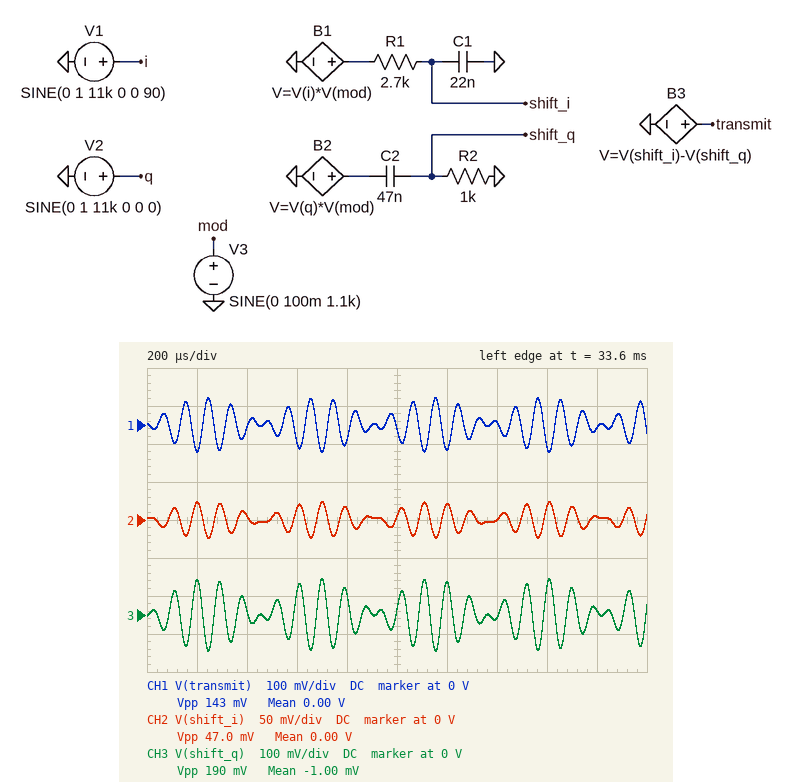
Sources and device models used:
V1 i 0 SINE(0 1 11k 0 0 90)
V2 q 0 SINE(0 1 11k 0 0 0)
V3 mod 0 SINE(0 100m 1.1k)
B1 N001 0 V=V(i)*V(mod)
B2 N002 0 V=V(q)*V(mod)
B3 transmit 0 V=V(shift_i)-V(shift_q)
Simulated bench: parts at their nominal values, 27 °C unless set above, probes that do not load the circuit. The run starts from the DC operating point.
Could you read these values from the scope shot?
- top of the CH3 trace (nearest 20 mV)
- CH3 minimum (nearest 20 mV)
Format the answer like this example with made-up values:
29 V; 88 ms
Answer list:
100 mV; -100 mV
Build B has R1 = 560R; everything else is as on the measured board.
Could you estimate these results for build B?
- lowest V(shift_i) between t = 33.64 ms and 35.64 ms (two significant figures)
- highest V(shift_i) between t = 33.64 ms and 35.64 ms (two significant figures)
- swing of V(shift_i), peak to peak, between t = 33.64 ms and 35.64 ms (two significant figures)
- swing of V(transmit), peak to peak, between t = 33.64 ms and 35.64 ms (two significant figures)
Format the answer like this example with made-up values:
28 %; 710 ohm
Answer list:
-76 mV; 76 mV; 150 mV; 100 mV
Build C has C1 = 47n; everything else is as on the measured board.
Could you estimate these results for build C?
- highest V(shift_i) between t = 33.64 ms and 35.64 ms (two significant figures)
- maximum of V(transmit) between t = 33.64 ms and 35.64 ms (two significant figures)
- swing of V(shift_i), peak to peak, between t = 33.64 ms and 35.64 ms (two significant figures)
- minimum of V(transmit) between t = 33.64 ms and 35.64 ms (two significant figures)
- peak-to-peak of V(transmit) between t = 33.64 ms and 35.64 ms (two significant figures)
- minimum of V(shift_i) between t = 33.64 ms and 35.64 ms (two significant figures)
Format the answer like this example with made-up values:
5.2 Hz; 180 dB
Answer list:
11 mV; 84 mV; 23 mV; -84 mV; 170 mV; -11 mV
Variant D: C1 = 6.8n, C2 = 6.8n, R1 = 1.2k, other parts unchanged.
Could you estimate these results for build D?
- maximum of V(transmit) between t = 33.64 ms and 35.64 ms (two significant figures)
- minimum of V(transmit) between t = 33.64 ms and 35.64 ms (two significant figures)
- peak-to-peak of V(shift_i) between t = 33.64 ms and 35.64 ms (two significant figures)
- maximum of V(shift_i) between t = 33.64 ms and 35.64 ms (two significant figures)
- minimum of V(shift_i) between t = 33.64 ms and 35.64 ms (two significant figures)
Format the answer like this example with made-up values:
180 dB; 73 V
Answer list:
45 mV; -45 mV; 170 mV; 87 mV; -87 mV
